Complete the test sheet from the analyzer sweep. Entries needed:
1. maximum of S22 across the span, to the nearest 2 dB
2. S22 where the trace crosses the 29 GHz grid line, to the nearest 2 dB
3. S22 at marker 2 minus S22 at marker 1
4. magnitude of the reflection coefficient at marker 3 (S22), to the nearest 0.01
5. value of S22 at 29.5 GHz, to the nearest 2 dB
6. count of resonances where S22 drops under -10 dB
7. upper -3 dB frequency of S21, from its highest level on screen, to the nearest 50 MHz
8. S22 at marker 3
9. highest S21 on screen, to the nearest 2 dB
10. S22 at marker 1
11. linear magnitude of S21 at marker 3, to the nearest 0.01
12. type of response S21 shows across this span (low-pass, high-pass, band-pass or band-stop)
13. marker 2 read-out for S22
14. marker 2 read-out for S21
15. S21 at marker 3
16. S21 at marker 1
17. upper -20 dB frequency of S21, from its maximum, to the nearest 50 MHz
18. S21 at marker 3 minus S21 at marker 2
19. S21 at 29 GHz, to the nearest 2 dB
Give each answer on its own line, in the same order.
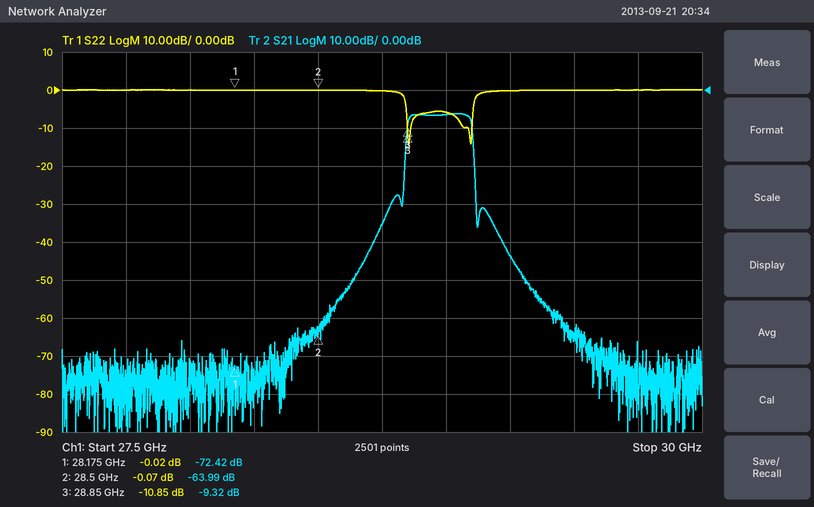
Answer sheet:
0 dB
-6 dB
-0.05 dB
0.29
0 dB
2
29.10 GHz
-10.85 dB
-6 dB
-0.02 dB
0.34
band-pass
-0.07 dB
-63.99 dB
-9.32 dB
-72.42 dB
29.10 GHz
54.67 dB
-6 dB
